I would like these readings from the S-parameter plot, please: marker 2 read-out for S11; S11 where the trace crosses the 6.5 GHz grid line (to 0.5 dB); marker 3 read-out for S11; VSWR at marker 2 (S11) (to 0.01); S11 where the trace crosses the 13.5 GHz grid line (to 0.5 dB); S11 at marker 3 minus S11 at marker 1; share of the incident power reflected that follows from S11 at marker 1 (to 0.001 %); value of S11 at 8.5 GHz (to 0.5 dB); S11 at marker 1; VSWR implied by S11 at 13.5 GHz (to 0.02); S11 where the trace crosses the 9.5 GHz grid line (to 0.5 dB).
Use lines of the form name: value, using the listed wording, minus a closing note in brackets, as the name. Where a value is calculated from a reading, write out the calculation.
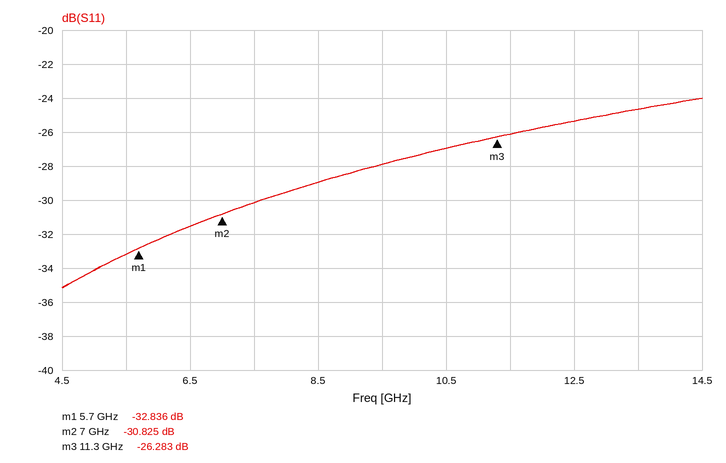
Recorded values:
marker 2 read-out for S11: -30.825 dB
S11 where the trace crosses the 6.5 GHz grid line: -31.5 dB
marker 3 read-out for S11: -26.283 dB
VSWR at marker 2 (S11): (1 + 0.0288)/(1 − 0.0288) ≈ 1.06
S11 where the trace crosses the 13.5 GHz grid line: -24.5 dB
S11 at marker 3 minus S11 at marker 1: -26.283 − (-32.836) = 6.553 dB
share of the incident power reflected that follows from S11 at marker 1: 10^(-32.836/10) ≈ 0.052 %
value of S11 at 8.5 GHz: -29.0 dB
S11 at marker 1: -32.836 dB
VSWR implied by S11 at 13.5 GHz: |Γ| = 10^(-24.5/20) = 0.0596; VSWR = (1 + 0.0596)/(1 − 0.0596) ≈ 1.13, so 1.12 to the nearest 0.02
S11 where the trace crosses the 9.5 GHz grid line: -28.0 dB
